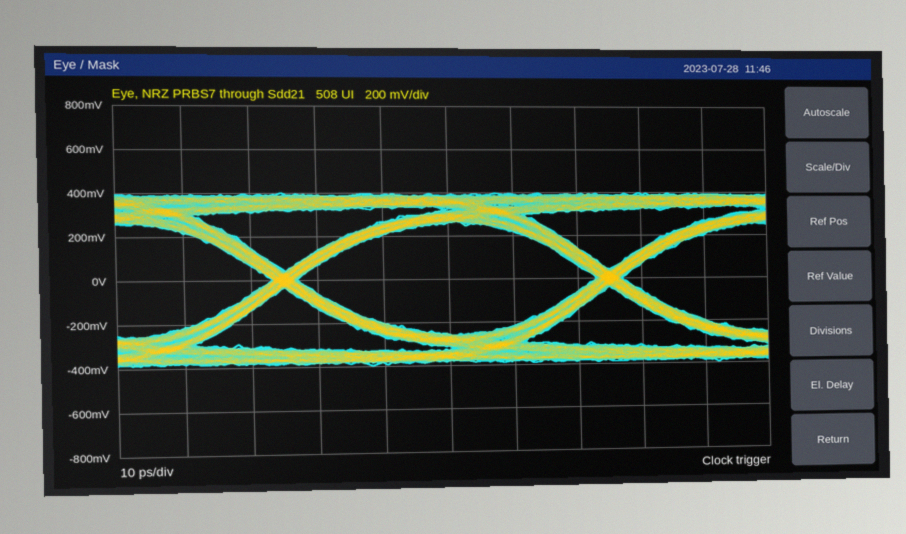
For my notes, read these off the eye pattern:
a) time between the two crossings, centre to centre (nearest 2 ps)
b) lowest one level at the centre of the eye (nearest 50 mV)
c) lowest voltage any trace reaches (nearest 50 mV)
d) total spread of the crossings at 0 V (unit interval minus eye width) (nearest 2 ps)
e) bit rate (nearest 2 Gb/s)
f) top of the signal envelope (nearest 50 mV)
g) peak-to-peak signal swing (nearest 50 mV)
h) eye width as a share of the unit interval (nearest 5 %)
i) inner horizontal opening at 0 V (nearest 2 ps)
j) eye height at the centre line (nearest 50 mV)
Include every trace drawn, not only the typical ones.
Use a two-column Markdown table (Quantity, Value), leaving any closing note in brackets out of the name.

| Quantity | Value |
|---|---|
| time between the two crossings, centre to centre | 50 ps |
| lowest one level at the centre of the eye | 250 mV |
| lowest voltage any trace reaches | -400 mV |
| total spread of the crossings at 0 V (unit interval minus eye width) | 4 ps |
| bit rate | 20 Gb/s |
| top of the signal envelope | 400 mV |
| peak-to-peak signal swing | 800 mV |
| eye width as a share of the unit interval | 90 % |
| inner horizontal opening at 0 V | 46 ps |
| eye height at the centre line | 500 mV |
